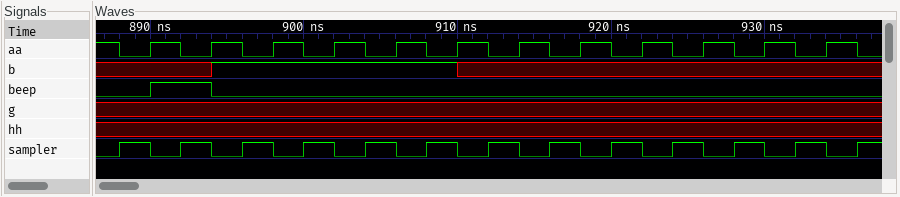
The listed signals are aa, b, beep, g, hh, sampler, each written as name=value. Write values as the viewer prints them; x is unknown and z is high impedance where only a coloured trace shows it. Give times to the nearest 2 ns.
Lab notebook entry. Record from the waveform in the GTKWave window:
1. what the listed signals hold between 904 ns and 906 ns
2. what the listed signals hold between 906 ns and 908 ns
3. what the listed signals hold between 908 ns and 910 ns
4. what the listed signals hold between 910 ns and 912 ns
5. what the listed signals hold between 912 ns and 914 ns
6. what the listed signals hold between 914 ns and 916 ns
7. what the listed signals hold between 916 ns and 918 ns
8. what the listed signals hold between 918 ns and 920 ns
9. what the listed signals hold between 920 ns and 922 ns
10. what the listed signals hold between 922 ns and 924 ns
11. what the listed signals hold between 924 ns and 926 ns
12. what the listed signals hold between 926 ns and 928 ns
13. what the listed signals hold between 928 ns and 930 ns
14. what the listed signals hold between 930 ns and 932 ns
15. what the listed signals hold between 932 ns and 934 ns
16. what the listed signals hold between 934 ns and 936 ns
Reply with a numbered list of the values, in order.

1. aa=0, b=1, beep=0, g=x, hh=x, sampler=1
2. aa=1, b=1, beep=0, g=x, hh=x, sampler=0
3. aa=0, b=1, beep=0, g=x, hh=x, sampler=1
4. aa=1, b=x, beep=0, g=x, hh=x, sampler=0
5. aa=0, b=x, beep=0, g=x, hh=x, sampler=1
6. aa=1, b=x, beep=0, g=x, hh=x, sampler=0
7. aa=0, b=x, beep=0, g=x, hh=x, sampler=1
8. aa=1, b=x, beep=0, g=x, hh=x, sampler=0
9. aa=0, b=x, beep=0, g=x, hh=x, sampler=1
10. aa=1, b=x, beep=0, g=x, hh=x, sampler=0
11. aa=0, b=x, beep=0, g=x, hh=x, sampler=1
12. aa=1, b=x, beep=0, g=x, hh=x, sampler=0
13. aa=0, b=x, beep=0, g=x, hh=x, sampler=1
14. aa=1, b=x, beep=0, g=x, hh=x, sampler=0
15. aa=0, b=x, beep=0, g=x, hh=x, sampler=1
16. aa=1, b=x, beep=0, g=x, hh=x, sampler=0
